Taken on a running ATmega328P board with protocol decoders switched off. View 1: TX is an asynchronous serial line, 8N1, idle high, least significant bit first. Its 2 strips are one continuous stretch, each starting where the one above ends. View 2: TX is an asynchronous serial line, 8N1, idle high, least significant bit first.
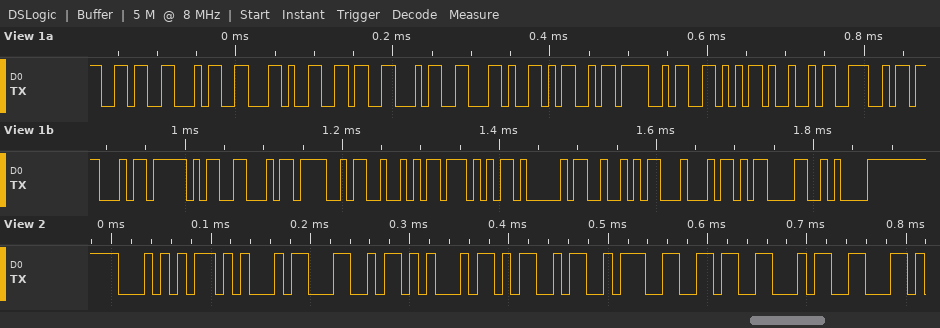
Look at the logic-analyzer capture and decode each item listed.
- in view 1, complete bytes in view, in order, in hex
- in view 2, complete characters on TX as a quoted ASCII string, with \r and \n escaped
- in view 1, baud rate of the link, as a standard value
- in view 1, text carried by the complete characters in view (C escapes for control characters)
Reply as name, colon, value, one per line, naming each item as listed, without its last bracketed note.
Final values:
in view 1, complete bytes in view, in order, in hex: 36 34 2C 36 34 2C 4D 4F 56 49 4E 47 5F 46 4F 52 57 41 52 44 0D 0A
in view 2, complete characters on TX as a quoted ASCII string, with \r and \n escaped: "TELEM:64"
in view 1, baud rate of the link, as a standard value: 115200 baud
in view 1, text carried by the complete characters in view: "64,64,MOVING_FORWARD\r\n"
